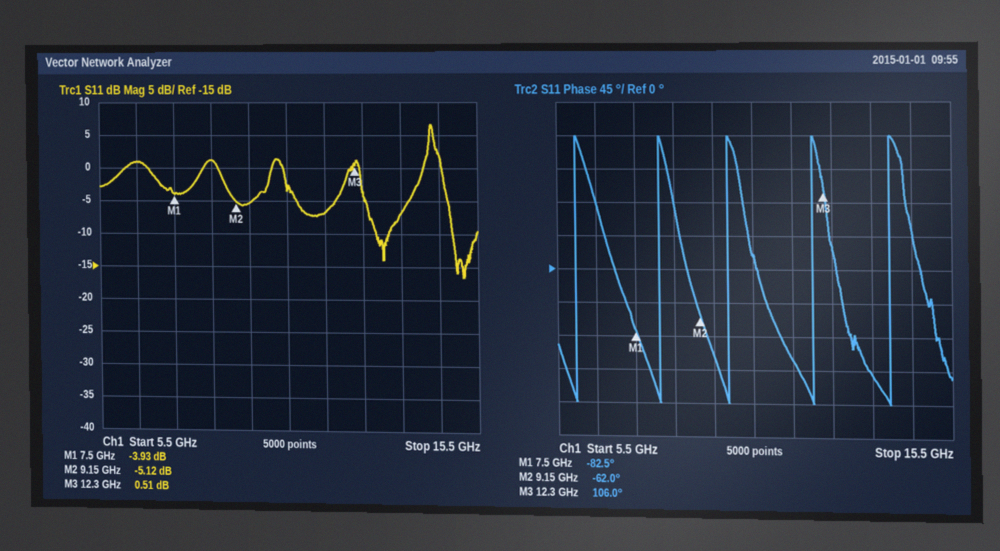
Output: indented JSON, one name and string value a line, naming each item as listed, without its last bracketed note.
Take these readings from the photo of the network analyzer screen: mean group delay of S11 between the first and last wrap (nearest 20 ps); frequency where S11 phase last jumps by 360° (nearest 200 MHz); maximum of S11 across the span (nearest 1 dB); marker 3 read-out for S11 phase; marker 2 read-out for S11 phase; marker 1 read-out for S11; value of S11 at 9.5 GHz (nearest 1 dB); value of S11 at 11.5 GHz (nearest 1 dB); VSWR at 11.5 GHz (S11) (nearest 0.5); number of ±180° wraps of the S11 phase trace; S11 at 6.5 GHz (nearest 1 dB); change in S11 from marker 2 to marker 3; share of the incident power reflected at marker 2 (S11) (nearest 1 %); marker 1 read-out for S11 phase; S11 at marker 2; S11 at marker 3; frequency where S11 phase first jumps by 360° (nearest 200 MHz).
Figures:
{
  "mean group delay of S11 between the first and last wrap": "500 ps",
  "frequency where S11 phase last jumps by 360°": "14.0 GHz",
  "maximum of S11 across the span": "7 dB",
  "marker 3 read-out for S11 phase": "106.0°",
  "marker 2 read-out for S11 phase": "-62.0°",
  "marker 1 read-out for S11": "-3.93 dB",
  "value of S11 at 9.5 GHz": "-5 dB",
  "value of S11 at 11.5 GHz": "-7 dB",
  "VSWR at 11.5 GHz (S11)": "2.5",
  "number of ±180° wraps of the S11 phase trace": "5",
  "S11 at 6.5 GHz": "1 dB",
  "change in S11 from marker 2 to marker 3": "5.63 dB",
  "share of the incident power reflected at marker 2 (S11)": "31 %",
  "marker 1 read-out for S11 phase": "-82.5°",
  "S11 at marker 2": "-5.12 dB",
  "S11 at marker 3": "0.51 dB",
  "frequency where S11 phase first jumps by 360°": "6.0 GHz"
}
